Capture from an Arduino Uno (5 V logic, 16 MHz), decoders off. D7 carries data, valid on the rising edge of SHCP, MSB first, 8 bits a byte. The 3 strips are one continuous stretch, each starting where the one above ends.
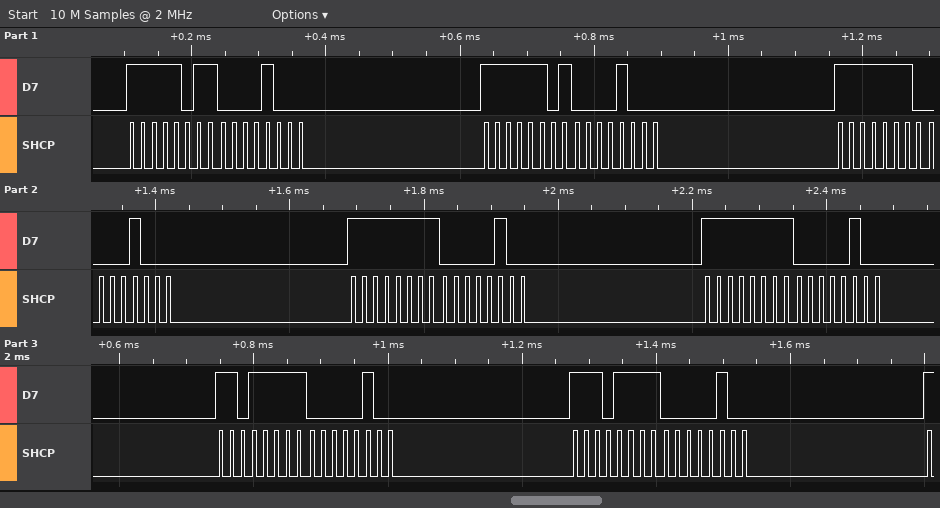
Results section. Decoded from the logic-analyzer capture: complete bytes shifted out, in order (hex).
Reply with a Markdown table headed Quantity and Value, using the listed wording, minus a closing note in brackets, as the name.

| Quantity | Value |
|---|---|
| complete bytes shifted out, in order | FB 08 FD 08 FE 08 FF 04 FF 04 DF 04 EF 04 |
